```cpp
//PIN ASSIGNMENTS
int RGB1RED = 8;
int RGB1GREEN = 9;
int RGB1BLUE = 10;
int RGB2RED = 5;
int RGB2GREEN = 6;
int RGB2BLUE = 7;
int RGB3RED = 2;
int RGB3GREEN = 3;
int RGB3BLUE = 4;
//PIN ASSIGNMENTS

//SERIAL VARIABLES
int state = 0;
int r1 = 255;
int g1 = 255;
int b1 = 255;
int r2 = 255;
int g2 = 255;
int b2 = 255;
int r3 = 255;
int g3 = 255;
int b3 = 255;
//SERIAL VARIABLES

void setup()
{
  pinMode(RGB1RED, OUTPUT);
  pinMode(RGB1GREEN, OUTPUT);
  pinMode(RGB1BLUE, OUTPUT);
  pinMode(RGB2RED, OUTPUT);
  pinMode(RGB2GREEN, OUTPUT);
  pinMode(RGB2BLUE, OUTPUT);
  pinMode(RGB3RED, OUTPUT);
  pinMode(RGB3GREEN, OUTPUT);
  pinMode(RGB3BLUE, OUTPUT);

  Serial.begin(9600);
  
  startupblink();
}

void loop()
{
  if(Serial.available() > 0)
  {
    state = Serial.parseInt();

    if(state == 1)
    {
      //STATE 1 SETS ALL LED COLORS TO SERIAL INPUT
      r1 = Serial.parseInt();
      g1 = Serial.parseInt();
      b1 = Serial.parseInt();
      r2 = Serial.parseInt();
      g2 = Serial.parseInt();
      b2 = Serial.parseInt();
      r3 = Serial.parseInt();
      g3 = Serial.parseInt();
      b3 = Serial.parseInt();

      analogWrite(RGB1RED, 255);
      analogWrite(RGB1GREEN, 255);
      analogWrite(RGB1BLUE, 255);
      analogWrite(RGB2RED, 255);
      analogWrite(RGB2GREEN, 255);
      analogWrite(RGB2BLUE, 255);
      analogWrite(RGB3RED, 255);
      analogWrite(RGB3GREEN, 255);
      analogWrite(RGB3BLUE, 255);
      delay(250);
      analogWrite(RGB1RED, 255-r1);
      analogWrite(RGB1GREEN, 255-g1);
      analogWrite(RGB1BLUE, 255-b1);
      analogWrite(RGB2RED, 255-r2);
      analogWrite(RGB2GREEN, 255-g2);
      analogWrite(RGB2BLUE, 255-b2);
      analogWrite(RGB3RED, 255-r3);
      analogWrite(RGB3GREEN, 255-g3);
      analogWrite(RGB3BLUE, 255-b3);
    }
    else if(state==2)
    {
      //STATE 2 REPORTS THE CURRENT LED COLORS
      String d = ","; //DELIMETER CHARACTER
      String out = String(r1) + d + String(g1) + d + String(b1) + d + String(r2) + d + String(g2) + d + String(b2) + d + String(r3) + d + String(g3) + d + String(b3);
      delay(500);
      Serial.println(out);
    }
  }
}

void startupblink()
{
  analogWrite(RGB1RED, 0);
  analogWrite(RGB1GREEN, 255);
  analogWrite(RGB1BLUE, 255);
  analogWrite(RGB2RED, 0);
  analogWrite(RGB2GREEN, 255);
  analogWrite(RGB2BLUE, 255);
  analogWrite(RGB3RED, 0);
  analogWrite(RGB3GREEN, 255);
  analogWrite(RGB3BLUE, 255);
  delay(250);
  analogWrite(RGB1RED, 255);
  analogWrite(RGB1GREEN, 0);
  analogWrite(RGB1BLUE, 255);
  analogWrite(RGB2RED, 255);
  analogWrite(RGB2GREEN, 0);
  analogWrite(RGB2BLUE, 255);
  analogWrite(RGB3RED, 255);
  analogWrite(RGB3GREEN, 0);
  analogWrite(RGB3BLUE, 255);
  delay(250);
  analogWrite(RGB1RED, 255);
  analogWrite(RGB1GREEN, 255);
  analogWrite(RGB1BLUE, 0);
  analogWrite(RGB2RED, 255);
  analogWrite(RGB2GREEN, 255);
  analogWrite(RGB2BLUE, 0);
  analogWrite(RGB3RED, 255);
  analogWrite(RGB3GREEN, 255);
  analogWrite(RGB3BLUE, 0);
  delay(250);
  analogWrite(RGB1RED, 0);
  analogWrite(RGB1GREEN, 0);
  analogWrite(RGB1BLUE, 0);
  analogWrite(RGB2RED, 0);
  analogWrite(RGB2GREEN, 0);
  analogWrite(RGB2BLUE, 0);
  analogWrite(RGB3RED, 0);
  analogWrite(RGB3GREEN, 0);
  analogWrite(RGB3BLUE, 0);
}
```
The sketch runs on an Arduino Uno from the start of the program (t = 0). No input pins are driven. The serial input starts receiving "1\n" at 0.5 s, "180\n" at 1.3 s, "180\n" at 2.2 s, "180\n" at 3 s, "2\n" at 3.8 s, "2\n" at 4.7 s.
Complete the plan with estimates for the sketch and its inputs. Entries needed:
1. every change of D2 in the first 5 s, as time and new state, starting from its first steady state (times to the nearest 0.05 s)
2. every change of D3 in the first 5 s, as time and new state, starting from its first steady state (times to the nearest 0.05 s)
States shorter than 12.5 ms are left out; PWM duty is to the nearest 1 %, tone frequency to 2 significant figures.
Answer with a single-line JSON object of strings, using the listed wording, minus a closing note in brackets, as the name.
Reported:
{"every change of D2 in the first 5 s, as time and new state, starting from its first steady state": "0 s low; 0.25 s high; 0.75 s low", "every change of D3 in the first 5 s, as time and new state, starting from its first steady state": "0 s high; 0.25 s low; 0.5 s high; 0.75 s low"}
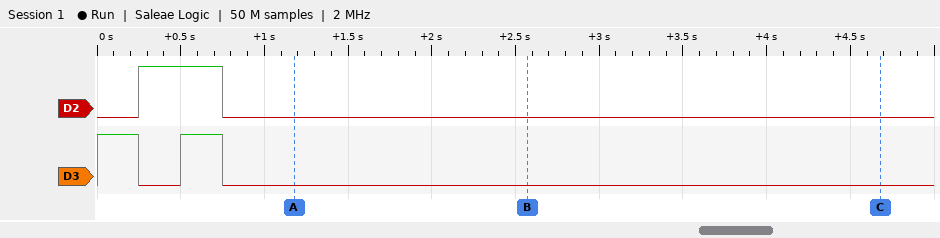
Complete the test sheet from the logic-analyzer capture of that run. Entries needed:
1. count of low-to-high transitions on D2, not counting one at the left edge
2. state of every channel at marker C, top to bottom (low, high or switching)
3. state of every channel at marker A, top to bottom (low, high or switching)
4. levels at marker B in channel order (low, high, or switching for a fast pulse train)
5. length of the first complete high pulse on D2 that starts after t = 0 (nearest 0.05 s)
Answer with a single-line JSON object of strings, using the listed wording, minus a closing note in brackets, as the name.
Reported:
{"count of low-to-high transitions on D2, not counting one at the left edge": "1", "state of every channel at marker C, top to bottom": "D2 low, D3 low", "state of every channel at marker A, top to bottom": "D2 low, D3 low", "levels at marker B in channel order": "D2 low, D3 low", "length of the first complete high pulse on D2 that starts after t = 0": "0.50 s"}
